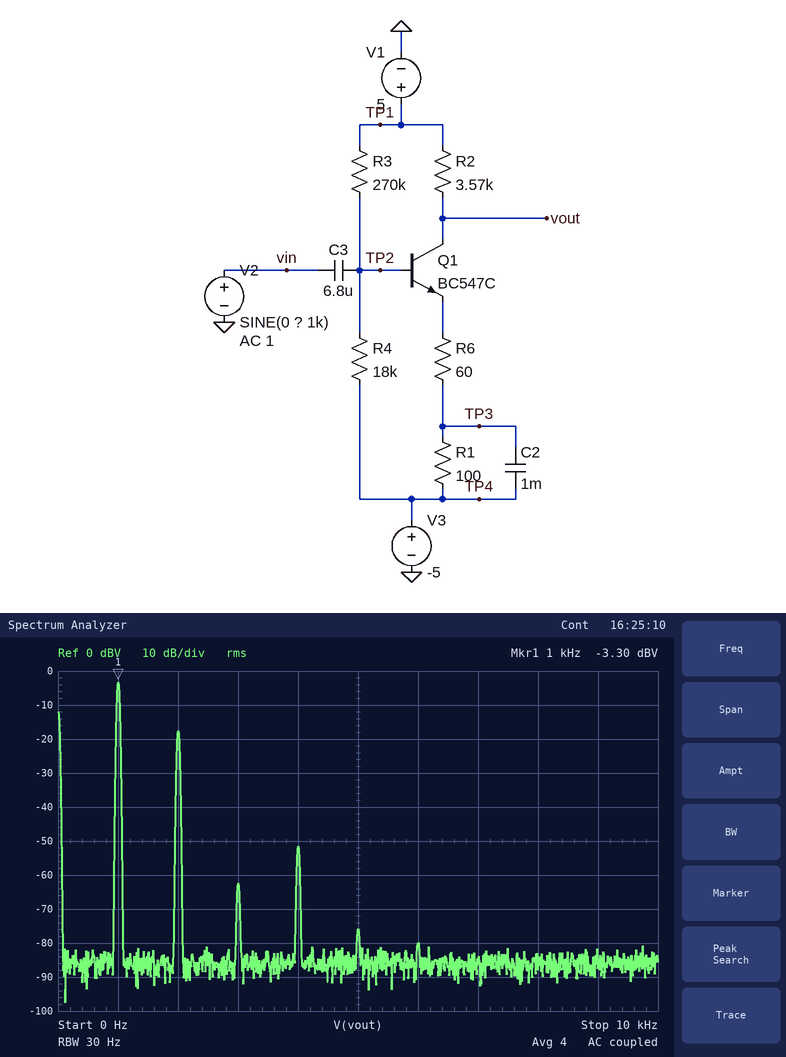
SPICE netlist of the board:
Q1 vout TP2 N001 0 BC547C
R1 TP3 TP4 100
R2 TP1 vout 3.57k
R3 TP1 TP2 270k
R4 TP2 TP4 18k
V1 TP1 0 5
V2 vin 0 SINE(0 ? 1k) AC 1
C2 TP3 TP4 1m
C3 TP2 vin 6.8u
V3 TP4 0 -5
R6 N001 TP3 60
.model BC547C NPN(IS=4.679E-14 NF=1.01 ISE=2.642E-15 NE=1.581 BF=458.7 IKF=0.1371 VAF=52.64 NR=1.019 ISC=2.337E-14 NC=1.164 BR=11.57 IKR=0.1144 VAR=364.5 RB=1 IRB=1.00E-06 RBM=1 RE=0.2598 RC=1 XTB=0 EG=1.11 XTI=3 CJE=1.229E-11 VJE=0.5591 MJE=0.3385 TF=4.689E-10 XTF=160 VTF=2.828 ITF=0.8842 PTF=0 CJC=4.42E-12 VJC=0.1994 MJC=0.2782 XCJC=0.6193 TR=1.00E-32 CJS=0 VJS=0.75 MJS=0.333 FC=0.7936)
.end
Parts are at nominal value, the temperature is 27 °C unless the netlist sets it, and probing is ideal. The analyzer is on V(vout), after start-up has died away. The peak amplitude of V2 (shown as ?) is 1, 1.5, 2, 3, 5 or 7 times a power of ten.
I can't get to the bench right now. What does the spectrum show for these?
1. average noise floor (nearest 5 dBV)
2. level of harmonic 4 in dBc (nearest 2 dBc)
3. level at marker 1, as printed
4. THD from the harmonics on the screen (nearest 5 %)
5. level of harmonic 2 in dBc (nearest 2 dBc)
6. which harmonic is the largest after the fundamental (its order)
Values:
-85 dBV
-48 dBc
-3.30 dBV
20 %
-14 dBc
2
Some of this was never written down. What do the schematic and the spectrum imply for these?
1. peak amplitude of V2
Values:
50 mV
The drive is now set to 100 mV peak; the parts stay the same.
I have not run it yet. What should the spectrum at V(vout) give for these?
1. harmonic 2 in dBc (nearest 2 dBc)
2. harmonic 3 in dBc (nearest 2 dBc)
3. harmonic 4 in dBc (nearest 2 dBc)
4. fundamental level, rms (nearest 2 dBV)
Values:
-10 dBc
-32 dBc
-34 dBc
2 dBV
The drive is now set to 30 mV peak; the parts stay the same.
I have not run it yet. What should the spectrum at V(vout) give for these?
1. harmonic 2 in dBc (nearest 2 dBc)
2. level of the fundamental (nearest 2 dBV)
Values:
-18 dBc
-8 dBV
